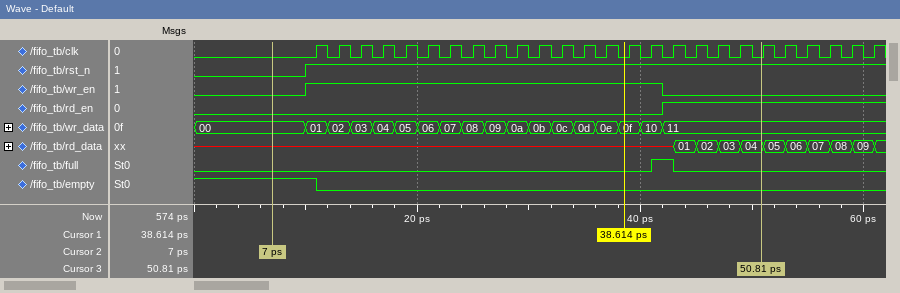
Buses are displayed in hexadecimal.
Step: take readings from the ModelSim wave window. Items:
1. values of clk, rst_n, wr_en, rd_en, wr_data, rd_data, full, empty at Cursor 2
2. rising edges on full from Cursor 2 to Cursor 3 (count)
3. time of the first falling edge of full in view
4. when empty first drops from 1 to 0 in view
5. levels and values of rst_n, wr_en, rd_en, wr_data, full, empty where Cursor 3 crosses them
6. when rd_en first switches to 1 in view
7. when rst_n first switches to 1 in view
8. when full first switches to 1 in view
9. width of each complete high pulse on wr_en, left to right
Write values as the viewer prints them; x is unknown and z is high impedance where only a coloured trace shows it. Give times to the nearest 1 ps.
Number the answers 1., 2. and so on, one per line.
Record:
1. clk=0, rst_n=0, wr_en=0, rd_en=0, wr_data=00, rd_data=x, full=0, empty=1
2. 1
3. 43 ps
4. 11 ps
5. rst_n=1, wr_en=0, rd_en=1, wr_data=11, full=0, empty=0
6. 42 ps
7. 10 ps
8. 41 ps
9. 32 ps
